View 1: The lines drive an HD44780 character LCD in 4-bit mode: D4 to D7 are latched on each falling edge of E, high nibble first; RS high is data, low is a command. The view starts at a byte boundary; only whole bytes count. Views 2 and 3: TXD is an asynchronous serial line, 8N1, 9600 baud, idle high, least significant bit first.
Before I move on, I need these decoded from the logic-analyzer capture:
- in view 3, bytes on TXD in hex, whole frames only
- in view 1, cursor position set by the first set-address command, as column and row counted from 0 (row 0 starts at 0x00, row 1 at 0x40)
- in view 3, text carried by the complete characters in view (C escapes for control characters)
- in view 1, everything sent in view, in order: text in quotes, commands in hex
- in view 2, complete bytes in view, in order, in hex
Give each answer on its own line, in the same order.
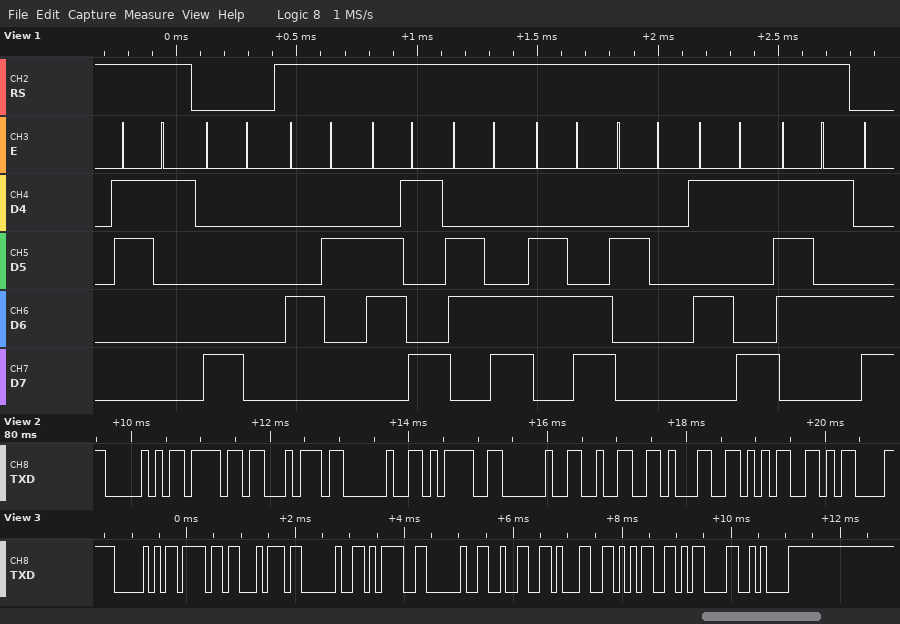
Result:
50 6F 74 20 3D 20 32 31 35 0D 0A
column 0, row 0
"Pot = 215\r\n"
"1" 0x80 "Bill Yu"
50 6F 74 20 3D 20 32 31 35 0D
